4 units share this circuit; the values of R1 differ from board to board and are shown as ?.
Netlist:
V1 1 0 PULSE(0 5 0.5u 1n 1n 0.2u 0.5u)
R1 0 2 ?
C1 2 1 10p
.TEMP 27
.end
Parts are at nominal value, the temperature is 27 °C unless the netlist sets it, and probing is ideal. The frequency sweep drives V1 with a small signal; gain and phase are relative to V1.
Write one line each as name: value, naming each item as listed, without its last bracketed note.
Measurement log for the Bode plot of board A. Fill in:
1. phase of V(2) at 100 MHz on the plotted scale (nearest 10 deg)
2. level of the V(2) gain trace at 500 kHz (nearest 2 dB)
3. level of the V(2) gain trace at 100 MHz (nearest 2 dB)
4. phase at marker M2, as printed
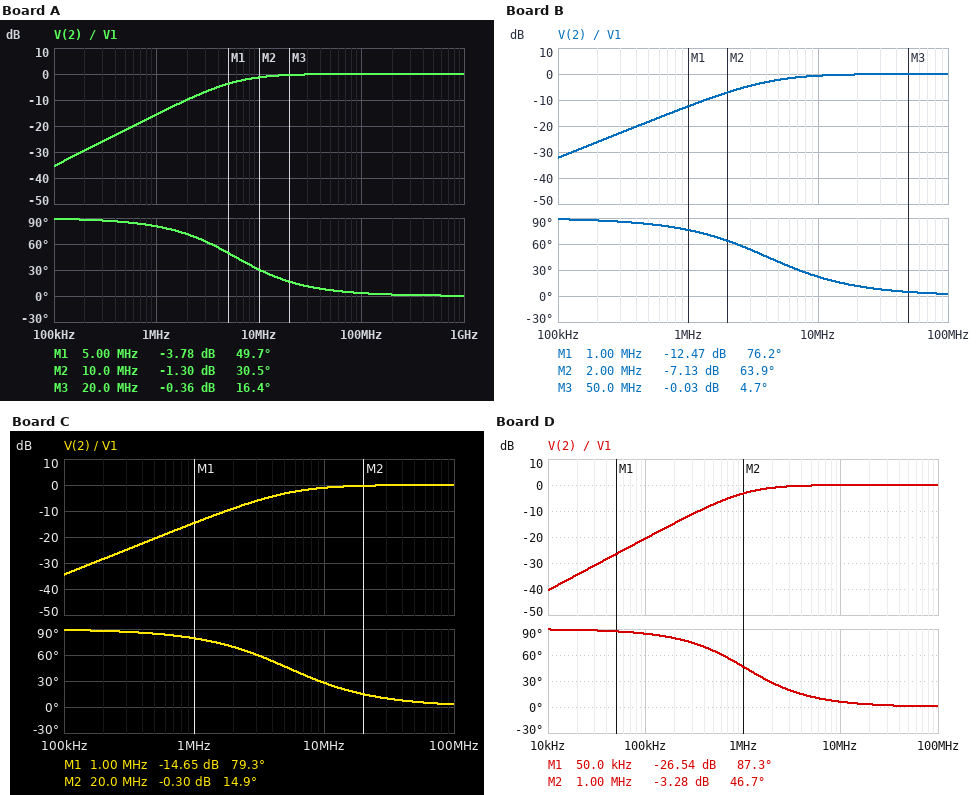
phase of V(2) at 100 MHz on the plotted scale: 0 deg
level of the V(2) gain trace at 500 kHz: -22 dB
level of the V(2) gain trace at 100 MHz: 0 dB
phase at marker M2, as printed: 30.5 deg
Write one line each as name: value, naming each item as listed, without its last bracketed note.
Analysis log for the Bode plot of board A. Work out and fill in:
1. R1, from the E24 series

R1, from the E24 series: 2.7 kΩ
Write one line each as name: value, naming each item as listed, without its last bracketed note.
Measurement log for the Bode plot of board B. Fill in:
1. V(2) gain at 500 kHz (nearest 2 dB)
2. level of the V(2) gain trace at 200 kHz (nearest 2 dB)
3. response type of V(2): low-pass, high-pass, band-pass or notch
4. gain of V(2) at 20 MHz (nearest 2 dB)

V(2) gain at 500 kHz: -18 dB
level of the V(2) gain trace at 200 kHz: -26 dB
response type of V(2): low-pass, high-pass, band-pass or notch: high-pass
gain of V(2) at 20 MHz: 0 dB
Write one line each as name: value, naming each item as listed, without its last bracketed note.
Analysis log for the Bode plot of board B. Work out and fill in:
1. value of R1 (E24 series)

value of R1: 3.9 kΩ
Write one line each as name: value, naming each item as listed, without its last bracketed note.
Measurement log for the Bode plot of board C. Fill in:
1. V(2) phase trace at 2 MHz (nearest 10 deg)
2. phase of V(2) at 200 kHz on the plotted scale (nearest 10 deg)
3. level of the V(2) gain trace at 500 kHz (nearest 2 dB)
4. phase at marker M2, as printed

V(2) phase trace at 2 MHz: 70 deg
phase of V(2) at 200 kHz on the plotted scale: 90 deg
level of the V(2) gain trace at 500 kHz: -20 dB
phase at marker M2, as printed: 14.9 deg
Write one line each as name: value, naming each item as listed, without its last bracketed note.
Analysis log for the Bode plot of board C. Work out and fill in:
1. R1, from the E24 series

R1, from the E24 series: 3 kΩ
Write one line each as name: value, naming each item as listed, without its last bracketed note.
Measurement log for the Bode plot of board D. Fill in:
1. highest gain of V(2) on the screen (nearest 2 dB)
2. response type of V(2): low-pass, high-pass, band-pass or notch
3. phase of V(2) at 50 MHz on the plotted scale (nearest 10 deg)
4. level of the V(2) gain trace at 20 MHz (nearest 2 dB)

highest gain of V(2) on the screen: 0 dB
response type of V(2): low-pass, high-pass, band-pass or notch: high-pass
phase of V(2) at 50 MHz on the plotted scale: 0 deg
level of the V(2) gain trace at 20 MHz: 0 dB
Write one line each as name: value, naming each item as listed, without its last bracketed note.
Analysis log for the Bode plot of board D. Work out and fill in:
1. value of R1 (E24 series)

value of R1: 15 kΩ
